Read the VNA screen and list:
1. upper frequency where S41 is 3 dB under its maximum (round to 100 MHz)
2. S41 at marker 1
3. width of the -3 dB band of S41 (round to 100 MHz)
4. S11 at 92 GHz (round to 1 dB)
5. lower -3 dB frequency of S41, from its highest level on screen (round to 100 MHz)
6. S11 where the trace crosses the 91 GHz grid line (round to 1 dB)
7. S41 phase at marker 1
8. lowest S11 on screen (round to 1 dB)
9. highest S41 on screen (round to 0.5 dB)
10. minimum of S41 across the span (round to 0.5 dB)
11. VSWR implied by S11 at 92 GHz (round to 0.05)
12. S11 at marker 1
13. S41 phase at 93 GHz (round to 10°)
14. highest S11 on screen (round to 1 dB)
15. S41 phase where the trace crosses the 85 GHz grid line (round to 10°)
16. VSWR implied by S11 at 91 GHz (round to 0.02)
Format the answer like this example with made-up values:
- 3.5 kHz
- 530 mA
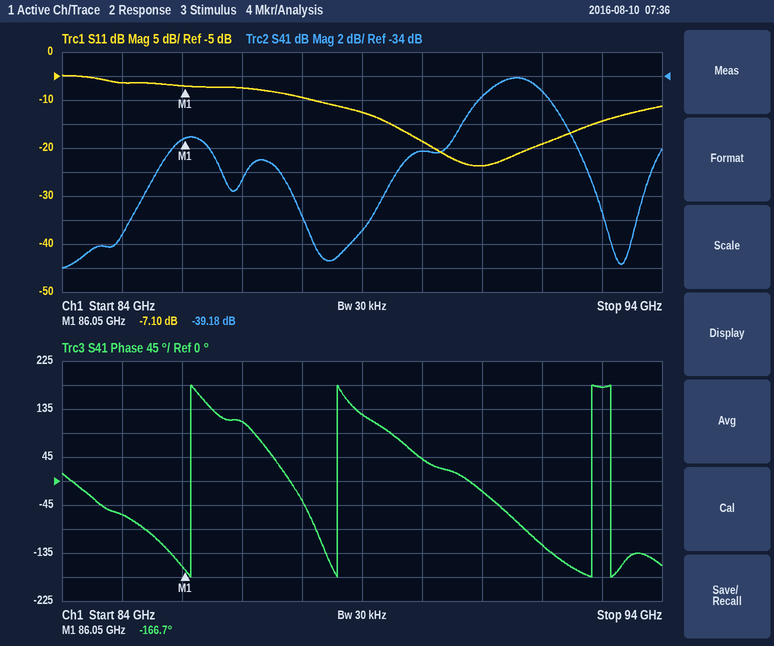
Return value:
- 92.3 GHz
- -39.18 dB
- 1.5 GHz
- -19 dB
- 90.8 GHz
- -24 dB
- -166.7°
- -24 dB
- -34.0 dB
- -50.0 dB
- 1.25
- -7.10 dB
- 180°
- -5 dB
- -60°
- 1.14
